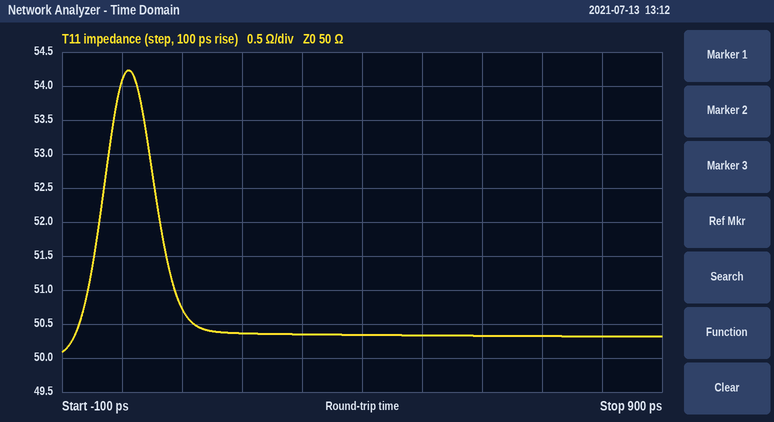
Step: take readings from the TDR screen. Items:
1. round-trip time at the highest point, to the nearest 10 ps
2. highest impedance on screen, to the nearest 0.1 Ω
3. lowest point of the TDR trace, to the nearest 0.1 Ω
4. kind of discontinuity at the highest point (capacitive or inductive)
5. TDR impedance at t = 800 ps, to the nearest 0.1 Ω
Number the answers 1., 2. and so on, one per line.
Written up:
1. 10 ps
2. 54.2 Ω
3. 50.1 Ω
4. inductive
5. 50.3 Ω
